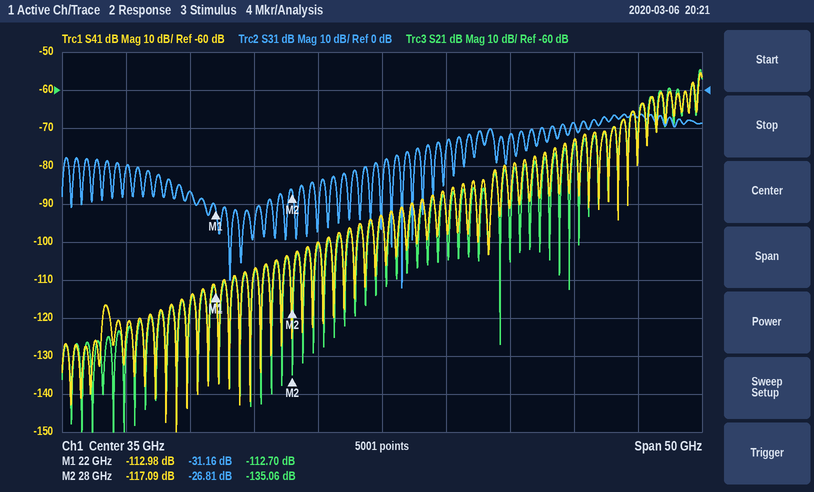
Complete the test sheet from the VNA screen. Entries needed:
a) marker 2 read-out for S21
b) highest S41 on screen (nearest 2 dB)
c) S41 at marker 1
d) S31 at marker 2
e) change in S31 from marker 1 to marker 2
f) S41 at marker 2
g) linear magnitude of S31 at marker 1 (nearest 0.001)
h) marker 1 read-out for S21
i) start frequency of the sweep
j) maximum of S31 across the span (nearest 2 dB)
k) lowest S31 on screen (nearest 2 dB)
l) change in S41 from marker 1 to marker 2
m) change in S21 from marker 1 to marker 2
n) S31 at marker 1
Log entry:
-135.06 dB
-56 dB
-112.98 dB
-26.81 dB
4.35 dB
-117.09 dB
0.028
-112.70 dB
10 GHz
-6 dB
-52 dB
-4.11 dB
-22.36 dB
-31.16 dB
